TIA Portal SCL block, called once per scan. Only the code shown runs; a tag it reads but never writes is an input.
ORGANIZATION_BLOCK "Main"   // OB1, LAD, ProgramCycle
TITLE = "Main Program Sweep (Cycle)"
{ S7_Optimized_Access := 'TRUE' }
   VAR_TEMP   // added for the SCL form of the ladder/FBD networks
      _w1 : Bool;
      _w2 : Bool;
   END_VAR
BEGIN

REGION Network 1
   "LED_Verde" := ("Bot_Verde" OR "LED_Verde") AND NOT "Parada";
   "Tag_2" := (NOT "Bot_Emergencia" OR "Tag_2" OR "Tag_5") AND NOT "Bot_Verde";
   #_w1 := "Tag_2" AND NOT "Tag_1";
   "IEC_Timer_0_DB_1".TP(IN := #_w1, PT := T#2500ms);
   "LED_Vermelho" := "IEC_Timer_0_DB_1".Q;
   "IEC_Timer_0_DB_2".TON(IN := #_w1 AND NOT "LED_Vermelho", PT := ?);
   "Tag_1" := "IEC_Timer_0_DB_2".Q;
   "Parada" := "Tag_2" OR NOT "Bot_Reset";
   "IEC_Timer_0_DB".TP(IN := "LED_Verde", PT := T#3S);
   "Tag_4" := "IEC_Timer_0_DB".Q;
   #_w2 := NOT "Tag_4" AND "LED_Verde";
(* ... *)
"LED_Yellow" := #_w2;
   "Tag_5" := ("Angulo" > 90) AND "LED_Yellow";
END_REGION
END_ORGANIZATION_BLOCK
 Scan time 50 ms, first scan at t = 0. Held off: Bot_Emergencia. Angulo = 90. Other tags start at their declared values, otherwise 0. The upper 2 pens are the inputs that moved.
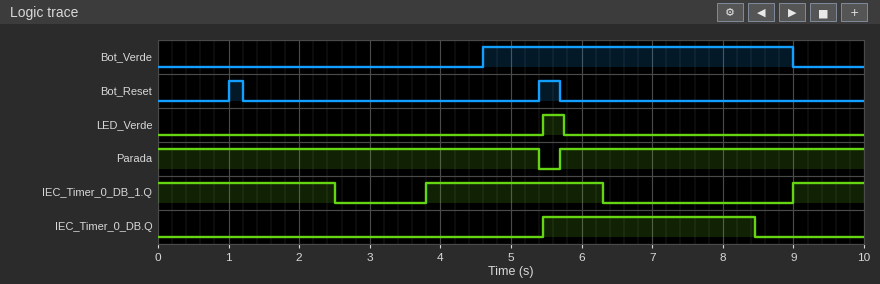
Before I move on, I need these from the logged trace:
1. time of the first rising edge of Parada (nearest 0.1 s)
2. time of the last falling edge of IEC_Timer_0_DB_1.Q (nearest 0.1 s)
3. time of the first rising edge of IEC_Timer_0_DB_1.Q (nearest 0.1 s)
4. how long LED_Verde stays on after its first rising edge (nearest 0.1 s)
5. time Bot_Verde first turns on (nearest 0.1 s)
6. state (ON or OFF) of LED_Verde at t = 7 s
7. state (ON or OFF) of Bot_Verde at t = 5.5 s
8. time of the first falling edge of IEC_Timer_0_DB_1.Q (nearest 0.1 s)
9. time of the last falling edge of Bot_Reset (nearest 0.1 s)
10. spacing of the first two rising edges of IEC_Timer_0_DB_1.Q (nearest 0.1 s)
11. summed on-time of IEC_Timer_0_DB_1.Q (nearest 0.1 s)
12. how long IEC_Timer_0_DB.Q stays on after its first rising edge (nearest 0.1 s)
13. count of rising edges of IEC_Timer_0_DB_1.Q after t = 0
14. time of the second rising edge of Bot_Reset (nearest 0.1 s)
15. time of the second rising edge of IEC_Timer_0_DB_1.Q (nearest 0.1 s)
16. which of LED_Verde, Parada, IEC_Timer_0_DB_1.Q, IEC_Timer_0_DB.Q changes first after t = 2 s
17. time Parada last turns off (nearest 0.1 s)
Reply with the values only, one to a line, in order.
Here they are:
5.7 s
6.3 s
3.8 s
0.3 s
4.6 s
OFF
ON
2.5 s
5.7 s
5.2 s
6.0 s
3.0 s
2
5.4 s
9.0 s
IEC_Timer_0_DB_1.Q
5.4 s
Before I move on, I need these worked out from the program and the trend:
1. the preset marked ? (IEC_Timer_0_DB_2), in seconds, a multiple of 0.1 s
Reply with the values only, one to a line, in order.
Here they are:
1.2 s
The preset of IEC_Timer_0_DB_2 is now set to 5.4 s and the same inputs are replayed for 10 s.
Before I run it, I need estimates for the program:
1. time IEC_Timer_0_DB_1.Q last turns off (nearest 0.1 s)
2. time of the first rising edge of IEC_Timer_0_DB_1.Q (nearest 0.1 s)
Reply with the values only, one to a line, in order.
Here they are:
2.5 s
9.0 s
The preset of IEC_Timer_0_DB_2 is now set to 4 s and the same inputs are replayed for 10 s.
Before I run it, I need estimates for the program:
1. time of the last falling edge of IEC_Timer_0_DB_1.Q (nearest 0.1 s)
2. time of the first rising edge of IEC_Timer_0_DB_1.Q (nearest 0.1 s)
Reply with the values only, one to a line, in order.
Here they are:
2.5 s
9.0 s
